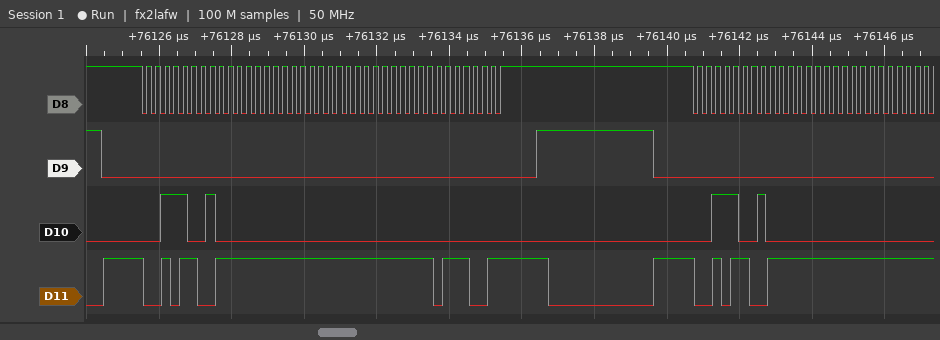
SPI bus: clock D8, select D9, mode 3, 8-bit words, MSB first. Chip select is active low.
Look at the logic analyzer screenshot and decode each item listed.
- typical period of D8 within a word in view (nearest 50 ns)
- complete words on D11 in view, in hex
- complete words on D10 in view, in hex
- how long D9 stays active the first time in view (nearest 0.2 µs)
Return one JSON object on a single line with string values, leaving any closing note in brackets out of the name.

{"typical period of D8 within a word in view": "250 ns", "complete words on D11 in view, in hex": "2C, FF, FF, FF, 73, 2C, FF, FF", "complete words on D10 in view, in hex": "39, 00, 00, 00, 00, 39, 00, 00", "how long D9 stays active the first time in view": "12 µs"}
